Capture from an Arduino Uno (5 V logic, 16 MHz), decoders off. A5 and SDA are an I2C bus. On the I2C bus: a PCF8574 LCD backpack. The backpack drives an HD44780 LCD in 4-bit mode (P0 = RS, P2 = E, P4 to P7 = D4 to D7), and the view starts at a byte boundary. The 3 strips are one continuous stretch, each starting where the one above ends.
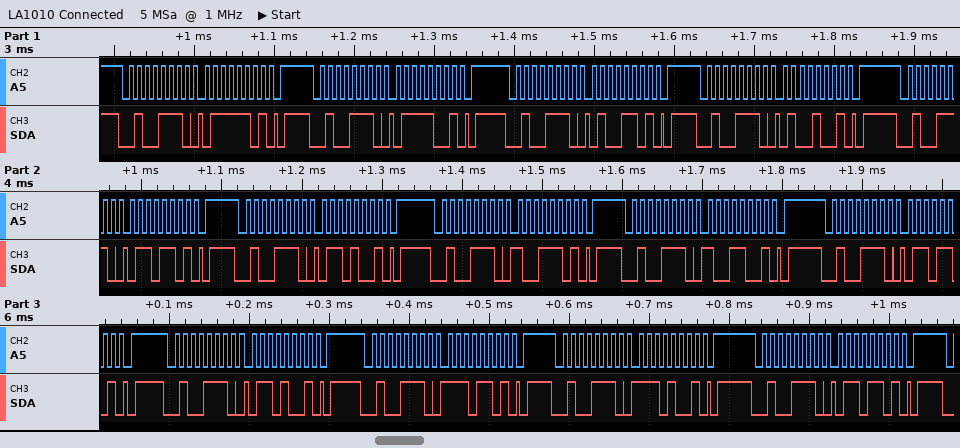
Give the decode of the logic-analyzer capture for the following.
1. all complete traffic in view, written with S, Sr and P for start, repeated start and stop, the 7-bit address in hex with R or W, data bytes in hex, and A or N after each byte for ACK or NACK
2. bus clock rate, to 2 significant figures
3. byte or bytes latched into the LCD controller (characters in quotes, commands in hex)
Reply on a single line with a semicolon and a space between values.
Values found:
S 27W A 7D A P S 27W A 79 A P S 27W A 4D A P S 27W A 49 A P S 27W A 6D A P S 27W A 69 A P S 27W A 9D A P S 27W A 99 A P S 27W A 6D A P S 27W A 69 A P S 27W A ED A P S 27W A E9 A P S 27W A 6D A P; 100 kHz; 't' 'i' 'n'
